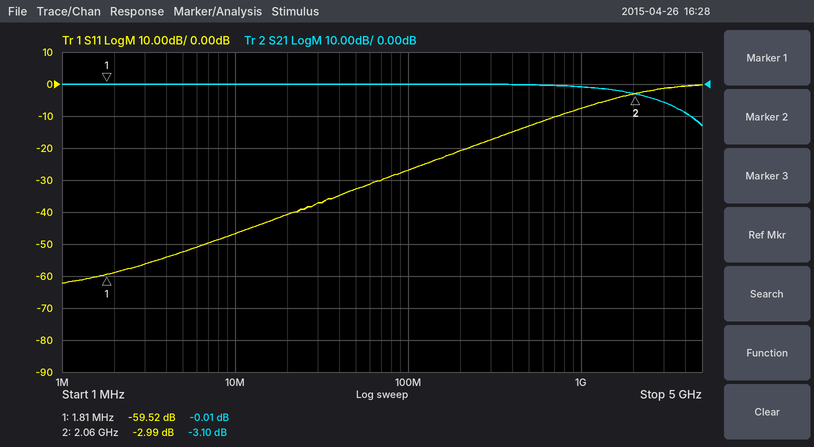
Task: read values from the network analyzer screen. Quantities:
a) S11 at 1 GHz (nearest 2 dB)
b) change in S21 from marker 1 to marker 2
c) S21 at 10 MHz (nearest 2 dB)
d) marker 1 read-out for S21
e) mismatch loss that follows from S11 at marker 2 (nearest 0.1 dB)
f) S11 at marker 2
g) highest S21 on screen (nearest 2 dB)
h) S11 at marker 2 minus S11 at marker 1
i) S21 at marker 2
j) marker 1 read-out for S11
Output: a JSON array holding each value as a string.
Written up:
["-8 dB", "-3.09 dB", "0 dB", "-0.01 dB", "3.0 dB", "-2.99 dB", "0 dB", "56.53 dB", "-3.10 dB", "-59.52 dB"]
